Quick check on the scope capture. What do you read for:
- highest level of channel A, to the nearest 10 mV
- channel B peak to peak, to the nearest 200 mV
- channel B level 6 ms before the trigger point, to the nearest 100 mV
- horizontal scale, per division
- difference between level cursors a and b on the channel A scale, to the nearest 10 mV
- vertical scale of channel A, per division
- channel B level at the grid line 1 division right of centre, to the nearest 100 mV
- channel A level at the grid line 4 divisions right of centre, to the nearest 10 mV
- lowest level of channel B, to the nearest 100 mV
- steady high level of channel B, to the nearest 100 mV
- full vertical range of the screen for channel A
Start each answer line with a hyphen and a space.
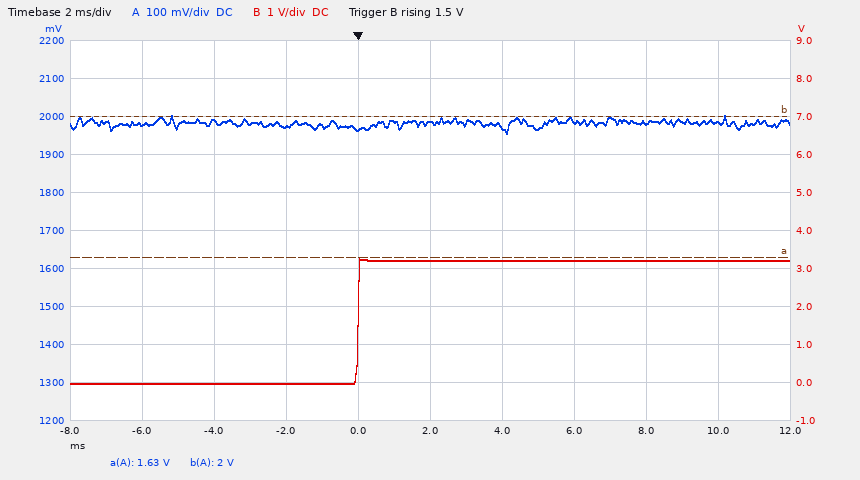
- 2.00 V
- 3.2 V
- 0.0 V
- 2 ms
- 370 mV
- 100 mV
- 3.2 V
- 1.98 V
- 0.0 V
- 3.2 V
- 1 V
